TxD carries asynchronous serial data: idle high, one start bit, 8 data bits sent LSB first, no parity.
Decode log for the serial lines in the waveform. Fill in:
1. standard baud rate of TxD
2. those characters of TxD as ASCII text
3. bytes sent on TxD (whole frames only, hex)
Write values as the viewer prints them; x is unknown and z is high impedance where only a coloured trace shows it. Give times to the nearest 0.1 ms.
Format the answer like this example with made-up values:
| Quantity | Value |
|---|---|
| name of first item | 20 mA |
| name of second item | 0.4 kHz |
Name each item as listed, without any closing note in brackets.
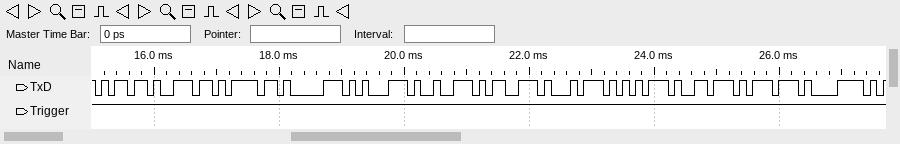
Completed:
| Quantity | Value |
|---|---|
| standard baud rate of TxD | 9600 baud |
| those characters of TxD as ASCII text | "mnopqrstuvwx" |
| bytes sent on TxD | 6D, 6E, 6F, 70, 71, 72, 73, 74, 75, 76, 77, 78 |
